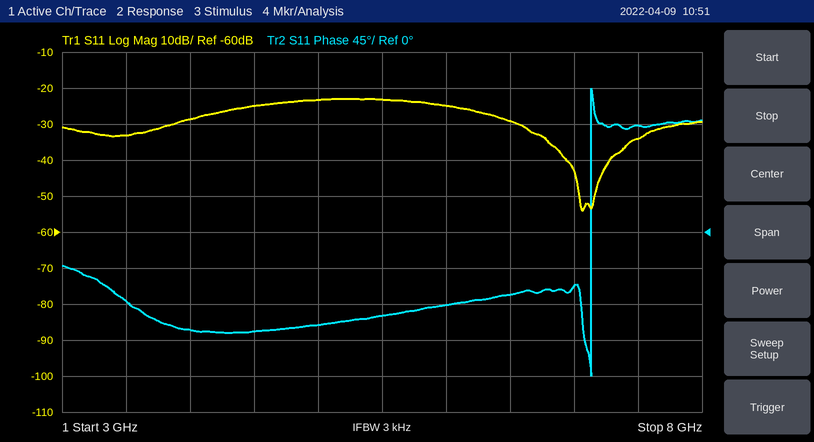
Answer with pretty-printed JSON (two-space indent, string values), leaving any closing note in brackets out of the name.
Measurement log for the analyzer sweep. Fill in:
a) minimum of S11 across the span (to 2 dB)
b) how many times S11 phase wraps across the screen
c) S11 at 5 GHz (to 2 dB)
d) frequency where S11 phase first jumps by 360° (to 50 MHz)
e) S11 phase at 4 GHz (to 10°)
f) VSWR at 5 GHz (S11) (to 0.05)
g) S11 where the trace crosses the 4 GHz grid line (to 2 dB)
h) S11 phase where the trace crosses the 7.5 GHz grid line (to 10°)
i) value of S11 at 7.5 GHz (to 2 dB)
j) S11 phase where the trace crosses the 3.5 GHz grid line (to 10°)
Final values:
{
  "minimum of S11 across the span": "-54 dB",
  "how many times S11 phase wraps across the screen": "1",
  "S11 at 5 GHz": "-24 dB",
  "frequency where S11 phase first jumps by 360°": "7.15 GHz",
  "S11 phase at 4 GHz": "-120°",
  "VSWR at 5 GHz (S11)": "1.15",
  "S11 where the trace crosses the 4 GHz grid line": "-28 dB",
  "S11 phase where the trace crosses the 7.5 GHz grid line": "130°",
  "value of S11 at 7.5 GHz": "-34 dB",
  "S11 phase where the trace crosses the 3.5 GHz grid line": "-90°"
}
